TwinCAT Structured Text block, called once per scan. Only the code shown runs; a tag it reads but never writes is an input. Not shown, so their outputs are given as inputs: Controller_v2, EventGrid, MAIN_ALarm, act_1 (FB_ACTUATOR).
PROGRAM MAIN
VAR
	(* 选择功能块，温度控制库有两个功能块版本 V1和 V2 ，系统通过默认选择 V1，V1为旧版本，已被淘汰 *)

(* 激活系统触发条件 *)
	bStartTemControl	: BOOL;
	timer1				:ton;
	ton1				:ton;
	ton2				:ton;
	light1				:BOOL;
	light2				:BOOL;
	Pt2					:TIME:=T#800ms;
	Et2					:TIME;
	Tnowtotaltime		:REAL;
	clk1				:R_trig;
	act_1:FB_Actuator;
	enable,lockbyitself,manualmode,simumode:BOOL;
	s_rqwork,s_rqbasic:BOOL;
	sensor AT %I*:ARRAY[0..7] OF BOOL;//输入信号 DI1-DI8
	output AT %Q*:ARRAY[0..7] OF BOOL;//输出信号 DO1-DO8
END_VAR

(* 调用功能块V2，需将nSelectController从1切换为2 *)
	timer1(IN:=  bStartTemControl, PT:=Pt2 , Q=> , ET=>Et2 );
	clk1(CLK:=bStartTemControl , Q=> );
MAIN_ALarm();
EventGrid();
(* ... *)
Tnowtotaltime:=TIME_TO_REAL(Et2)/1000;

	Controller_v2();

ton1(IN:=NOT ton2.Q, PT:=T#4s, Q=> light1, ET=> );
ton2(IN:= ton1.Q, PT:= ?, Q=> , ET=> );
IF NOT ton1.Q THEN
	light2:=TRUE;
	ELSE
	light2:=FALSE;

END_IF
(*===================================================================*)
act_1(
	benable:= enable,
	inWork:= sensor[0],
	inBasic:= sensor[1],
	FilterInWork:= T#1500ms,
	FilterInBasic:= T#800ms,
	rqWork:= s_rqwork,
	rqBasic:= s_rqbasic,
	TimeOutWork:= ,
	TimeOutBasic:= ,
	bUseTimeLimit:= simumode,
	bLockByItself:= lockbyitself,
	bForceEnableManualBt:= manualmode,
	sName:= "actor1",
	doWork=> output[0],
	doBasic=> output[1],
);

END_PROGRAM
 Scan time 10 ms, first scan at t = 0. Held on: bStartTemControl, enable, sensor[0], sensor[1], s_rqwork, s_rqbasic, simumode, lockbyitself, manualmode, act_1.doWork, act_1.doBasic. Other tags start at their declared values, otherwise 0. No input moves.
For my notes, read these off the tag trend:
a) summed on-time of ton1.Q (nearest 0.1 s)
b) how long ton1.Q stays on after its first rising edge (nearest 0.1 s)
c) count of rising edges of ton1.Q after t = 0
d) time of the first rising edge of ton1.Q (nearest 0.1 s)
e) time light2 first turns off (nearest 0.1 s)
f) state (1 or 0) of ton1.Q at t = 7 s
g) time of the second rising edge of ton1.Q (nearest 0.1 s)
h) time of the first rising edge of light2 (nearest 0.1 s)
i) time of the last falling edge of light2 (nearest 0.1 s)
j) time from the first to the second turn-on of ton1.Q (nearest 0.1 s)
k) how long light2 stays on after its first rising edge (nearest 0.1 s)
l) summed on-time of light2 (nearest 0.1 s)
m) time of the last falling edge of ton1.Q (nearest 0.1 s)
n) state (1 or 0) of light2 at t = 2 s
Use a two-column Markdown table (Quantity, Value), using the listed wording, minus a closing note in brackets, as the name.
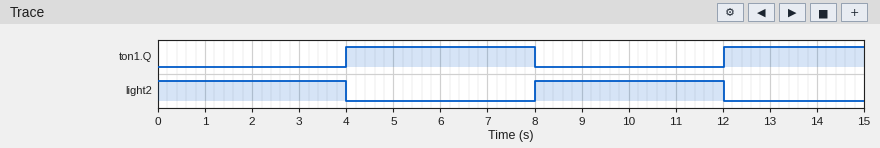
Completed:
| Quantity | Value |
|---|---|
| summed on-time of ton1.Q | 7.0 s |
| how long ton1.Q stays on after its first rising edge | 4.0 s |
| count of rising edges of ton1.Q after t = 0 | 2 |
| time of the first rising edge of ton1.Q | 4.0 s |
| time light2 first turns off | 4.0 s |
| state (1 or 0) of ton1.Q at t = 7 s | 1 |
| time of the second rising edge of ton1.Q | 12.0 s |
| time of the first rising edge of light2 | 8.0 s |
| time of the last falling edge of light2 | 12.0 s |
| time from the first to the second turn-on of ton1.Q | 8.0 s |
| how long light2 stays on after its first rising edge | 4.0 s |
| summed on-time of light2 | 8.0 s |
| time of the last falling edge of ton1.Q | 8.0 s |
| state (1 or 0) of light2 at t = 2 s | 1 |
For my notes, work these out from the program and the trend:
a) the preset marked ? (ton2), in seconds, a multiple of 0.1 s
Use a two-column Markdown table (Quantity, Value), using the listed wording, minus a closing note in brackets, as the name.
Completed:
| Quantity | Value |
|---|---|
| the preset marked ? (ton2), in seconds, a multiple of 0.1 s | 4.0 s |
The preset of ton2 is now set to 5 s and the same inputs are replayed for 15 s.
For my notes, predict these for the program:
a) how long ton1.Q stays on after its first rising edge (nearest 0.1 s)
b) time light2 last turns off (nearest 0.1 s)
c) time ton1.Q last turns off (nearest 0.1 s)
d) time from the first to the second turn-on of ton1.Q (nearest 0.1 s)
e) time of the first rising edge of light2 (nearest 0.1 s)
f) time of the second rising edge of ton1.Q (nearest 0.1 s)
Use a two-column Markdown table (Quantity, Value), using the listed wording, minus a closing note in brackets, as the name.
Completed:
| Quantity | Value |
|---|---|
| how long ton1.Q stays on after its first rising edge | 5.0 s |
| time light2 last turns off | 13.0 s |
| time ton1.Q last turns off | 9.0 s |
| time from the first to the second turn-on of ton1.Q | 9.0 s |
| time of the first rising edge of light2 | 9.0 s |
| time of the second rising edge of ton1.Q | 13.0 s |
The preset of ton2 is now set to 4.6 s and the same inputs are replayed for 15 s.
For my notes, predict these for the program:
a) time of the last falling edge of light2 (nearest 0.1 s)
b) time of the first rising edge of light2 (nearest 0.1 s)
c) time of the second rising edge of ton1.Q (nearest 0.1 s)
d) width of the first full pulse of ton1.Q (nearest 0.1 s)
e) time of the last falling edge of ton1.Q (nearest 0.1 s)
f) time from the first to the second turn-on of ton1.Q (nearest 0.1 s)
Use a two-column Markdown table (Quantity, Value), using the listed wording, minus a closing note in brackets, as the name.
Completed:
| Quantity | Value |
|---|---|
| time of the last falling edge of light2 | 12.6 s |
| time of the first rising edge of light2 | 8.6 s |
| time of the second rising edge of ton1.Q | 12.6 s |
| width of the first full pulse of ton1.Q | 4.6 s |
| time of the last falling edge of ton1.Q | 8.6 s |
| time from the first to the second turn-on of ton1.Q | 8.6 s |
